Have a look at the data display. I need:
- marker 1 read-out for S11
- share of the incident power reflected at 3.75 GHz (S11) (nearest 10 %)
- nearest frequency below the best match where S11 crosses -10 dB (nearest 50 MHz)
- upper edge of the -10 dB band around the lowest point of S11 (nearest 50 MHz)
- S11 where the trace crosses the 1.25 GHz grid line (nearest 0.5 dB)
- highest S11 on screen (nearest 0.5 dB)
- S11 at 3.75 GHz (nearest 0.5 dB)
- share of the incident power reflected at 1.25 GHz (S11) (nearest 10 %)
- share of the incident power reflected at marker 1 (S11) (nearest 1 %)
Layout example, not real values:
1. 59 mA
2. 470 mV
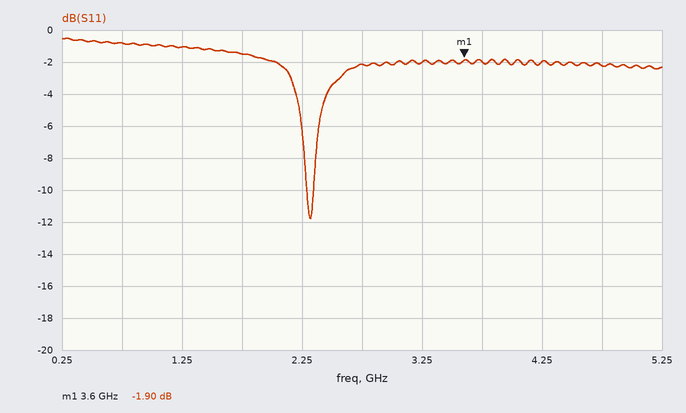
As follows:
1. -1.90 dB
2. 60 %
3. 2.30 GHz
4. 2.35 GHz
5. -1.0 dB
6. -0.5 dB
7. -2.0 dB
8. 80 %
9. 65 %
